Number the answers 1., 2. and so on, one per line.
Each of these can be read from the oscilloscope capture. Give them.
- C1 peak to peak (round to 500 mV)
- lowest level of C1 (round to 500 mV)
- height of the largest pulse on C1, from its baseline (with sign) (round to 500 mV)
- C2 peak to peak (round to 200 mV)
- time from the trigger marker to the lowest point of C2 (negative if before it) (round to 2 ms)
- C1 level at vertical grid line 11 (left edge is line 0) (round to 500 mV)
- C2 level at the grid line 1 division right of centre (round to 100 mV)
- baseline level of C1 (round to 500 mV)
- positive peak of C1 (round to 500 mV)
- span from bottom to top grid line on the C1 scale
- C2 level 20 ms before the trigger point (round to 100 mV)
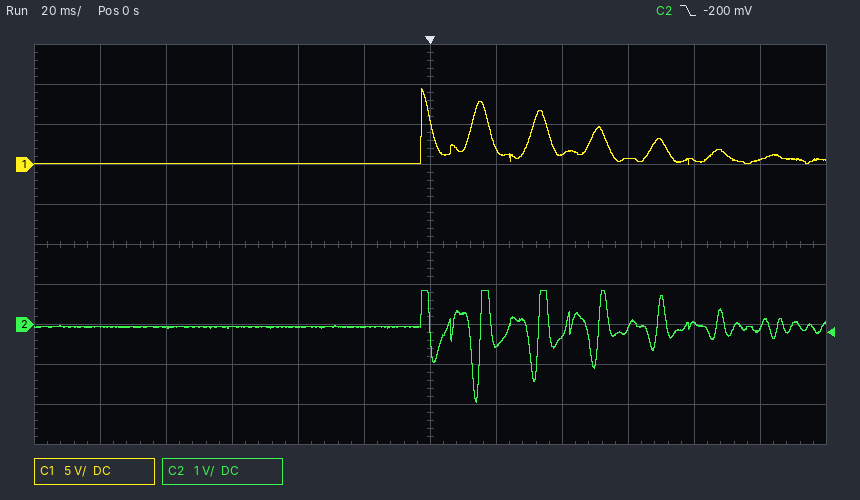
1. 9.5 V
2. 0.0 V
3. +9.5 V
4. 2.8 V
5. +14 ms
6. 500 mV
7. -500 mV
8. 0.0 V
9. 9.5 V
10. 50 V
11. -100 mV
